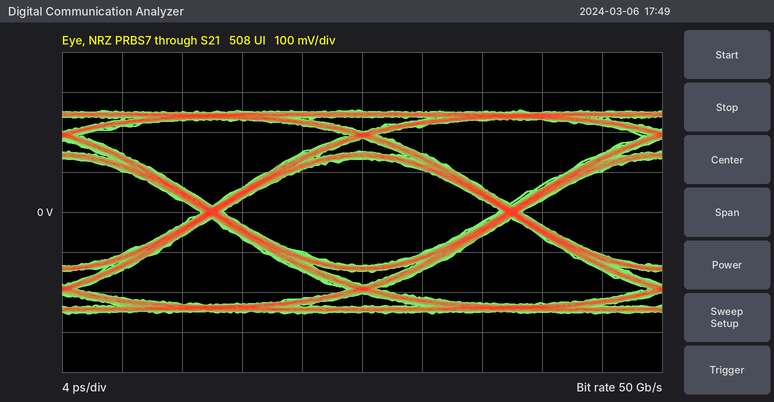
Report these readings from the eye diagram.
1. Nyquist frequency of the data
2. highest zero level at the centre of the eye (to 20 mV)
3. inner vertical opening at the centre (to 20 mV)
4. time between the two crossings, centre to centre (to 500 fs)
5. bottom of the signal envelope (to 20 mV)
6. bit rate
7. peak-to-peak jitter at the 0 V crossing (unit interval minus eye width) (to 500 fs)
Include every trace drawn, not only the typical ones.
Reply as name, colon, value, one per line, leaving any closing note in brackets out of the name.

Nyquist frequency of the data: 25 GHz
highest zero level at the centre of the eye: -140 mV
inner vertical opening at the centre: 260 mV
time between the two crossings, centre to centre: 20.0 ps
bottom of the signal envelope: -260 mV
bit rate: 50 Gb/s
peak-to-peak jitter at the 0 V crossing (unit interval minus eye width): 1.5 ps
